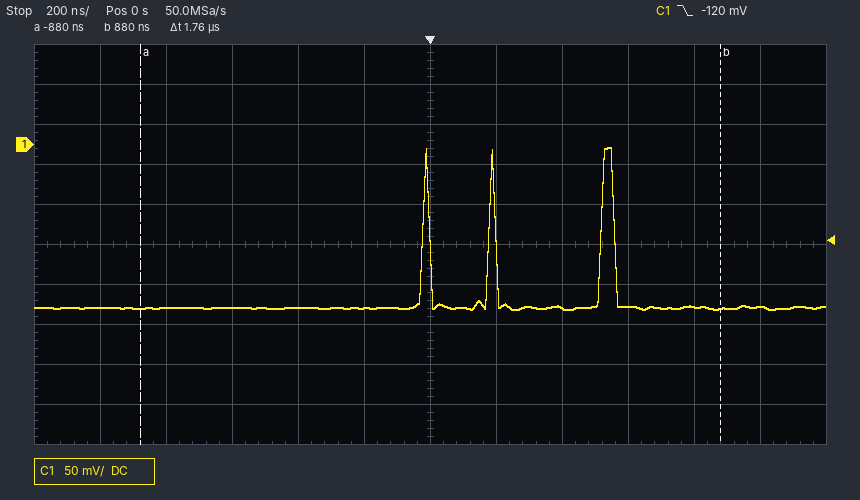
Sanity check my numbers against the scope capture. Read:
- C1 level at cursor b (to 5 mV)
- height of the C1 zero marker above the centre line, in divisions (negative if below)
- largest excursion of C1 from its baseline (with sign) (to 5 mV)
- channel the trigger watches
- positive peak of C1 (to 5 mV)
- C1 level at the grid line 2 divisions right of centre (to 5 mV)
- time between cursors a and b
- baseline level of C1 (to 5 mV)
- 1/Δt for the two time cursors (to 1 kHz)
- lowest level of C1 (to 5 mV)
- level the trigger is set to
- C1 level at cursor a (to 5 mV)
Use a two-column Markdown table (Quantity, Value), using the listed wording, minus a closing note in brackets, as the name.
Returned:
| Quantity | Value |
|---|---|
| C1 level at cursor b | -205 mV |
| height of the C1 zero marker above the centre line, in divisions | +2.5 div |
| largest excursion of C1 from its baseline (with sign) | +200 mV |
| channel the trigger watches | C1 |
| positive peak of C1 | -5 mV |
| C1 level at the grid line 2 divisions right of centre | -205 mV |
| time between cursors a and b | 1.76 µs |
| baseline level of C1 | -205 mV |
| 1/Δt for the two time cursors | 568 kHz |
| lowest level of C1 | -205 mV |
| level the trigger is set to | -120 mV |
| C1 level at cursor a | -205 mV |
